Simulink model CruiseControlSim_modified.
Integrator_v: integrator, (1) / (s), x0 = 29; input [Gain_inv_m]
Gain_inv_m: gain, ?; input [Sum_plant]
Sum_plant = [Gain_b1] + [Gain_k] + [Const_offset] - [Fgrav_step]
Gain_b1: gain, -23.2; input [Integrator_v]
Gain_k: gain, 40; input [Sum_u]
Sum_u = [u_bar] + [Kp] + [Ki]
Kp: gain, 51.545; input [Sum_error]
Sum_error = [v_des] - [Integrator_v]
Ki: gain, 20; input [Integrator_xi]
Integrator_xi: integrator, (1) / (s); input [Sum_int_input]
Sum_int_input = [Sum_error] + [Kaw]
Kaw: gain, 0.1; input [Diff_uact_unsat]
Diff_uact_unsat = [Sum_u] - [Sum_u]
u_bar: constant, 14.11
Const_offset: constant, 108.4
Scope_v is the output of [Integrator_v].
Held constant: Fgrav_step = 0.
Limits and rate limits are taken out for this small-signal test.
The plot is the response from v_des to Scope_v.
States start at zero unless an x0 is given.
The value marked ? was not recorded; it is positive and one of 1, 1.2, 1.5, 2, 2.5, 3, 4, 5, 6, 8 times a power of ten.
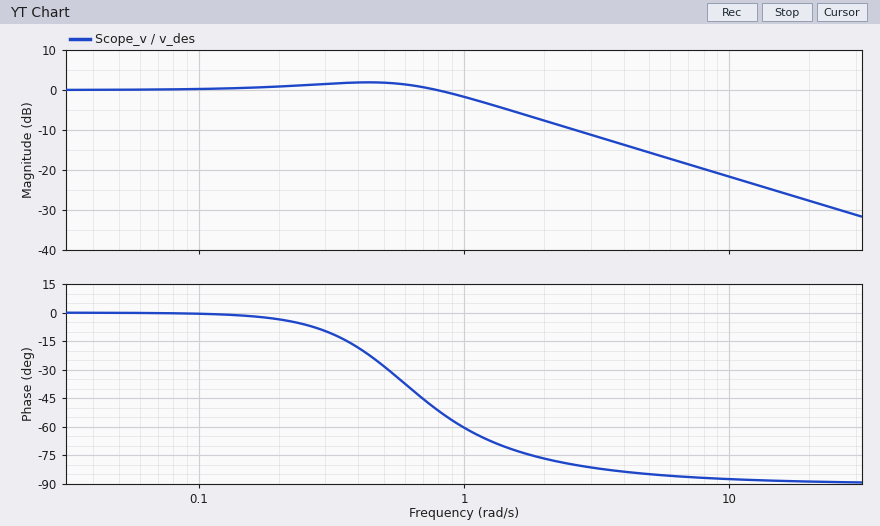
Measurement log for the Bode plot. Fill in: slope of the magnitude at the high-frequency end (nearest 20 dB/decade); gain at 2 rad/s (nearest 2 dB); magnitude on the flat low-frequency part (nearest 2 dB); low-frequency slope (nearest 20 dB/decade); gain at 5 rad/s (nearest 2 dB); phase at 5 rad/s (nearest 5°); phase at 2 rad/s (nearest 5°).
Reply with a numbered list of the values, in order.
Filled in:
1. -20 dB/decade
2. -8 dB
3. 0 dB
4. 0 dB/decade
5. -16 dB
6. -85°
7. -75°
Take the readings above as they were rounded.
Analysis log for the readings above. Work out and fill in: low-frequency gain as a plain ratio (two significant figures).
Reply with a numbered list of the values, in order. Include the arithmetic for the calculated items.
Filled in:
1. 10^(0 / 20) = 1.0
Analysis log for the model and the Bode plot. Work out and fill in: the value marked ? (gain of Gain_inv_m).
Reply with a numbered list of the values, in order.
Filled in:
1. 0.0004
